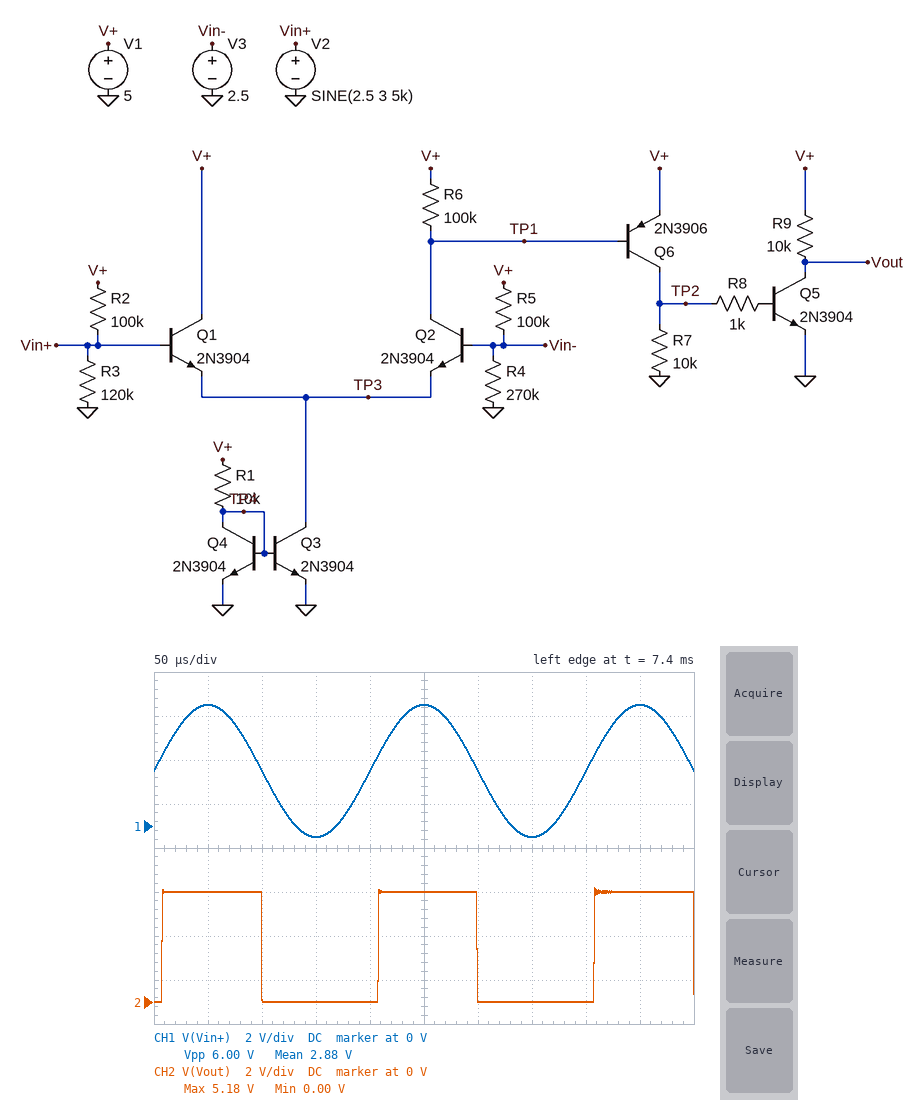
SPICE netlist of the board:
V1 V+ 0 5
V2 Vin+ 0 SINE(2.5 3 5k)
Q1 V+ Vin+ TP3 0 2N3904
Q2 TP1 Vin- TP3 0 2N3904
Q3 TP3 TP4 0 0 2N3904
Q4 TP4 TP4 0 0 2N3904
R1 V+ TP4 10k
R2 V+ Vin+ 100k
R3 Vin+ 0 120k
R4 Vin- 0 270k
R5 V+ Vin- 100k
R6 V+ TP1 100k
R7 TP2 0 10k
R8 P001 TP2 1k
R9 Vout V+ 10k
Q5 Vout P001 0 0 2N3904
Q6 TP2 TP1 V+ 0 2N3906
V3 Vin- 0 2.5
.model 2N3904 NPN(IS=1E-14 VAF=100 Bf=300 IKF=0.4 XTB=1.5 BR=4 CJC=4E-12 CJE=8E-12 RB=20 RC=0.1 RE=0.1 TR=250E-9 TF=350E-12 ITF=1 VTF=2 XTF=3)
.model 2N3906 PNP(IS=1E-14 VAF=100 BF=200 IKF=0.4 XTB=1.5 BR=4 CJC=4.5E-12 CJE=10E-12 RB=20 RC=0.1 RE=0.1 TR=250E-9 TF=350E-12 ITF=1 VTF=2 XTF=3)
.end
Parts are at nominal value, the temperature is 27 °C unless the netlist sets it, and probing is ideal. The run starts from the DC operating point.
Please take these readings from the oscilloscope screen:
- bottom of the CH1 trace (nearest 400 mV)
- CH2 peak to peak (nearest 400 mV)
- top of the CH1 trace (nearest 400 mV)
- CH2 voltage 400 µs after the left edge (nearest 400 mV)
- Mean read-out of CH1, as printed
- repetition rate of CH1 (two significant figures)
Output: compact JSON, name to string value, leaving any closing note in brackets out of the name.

{"bottom of the CH1 trace": "-400 mV", "CH2 peak to peak": "5.2 V", "top of the CH1 trace": "5.6 V", "CH2 voltage 400 µs after the left edge": "0 V", "Mean read-out of CH1, as printed": "2.88 V", "repetition rate of CH1": "5.0 kHz"}
